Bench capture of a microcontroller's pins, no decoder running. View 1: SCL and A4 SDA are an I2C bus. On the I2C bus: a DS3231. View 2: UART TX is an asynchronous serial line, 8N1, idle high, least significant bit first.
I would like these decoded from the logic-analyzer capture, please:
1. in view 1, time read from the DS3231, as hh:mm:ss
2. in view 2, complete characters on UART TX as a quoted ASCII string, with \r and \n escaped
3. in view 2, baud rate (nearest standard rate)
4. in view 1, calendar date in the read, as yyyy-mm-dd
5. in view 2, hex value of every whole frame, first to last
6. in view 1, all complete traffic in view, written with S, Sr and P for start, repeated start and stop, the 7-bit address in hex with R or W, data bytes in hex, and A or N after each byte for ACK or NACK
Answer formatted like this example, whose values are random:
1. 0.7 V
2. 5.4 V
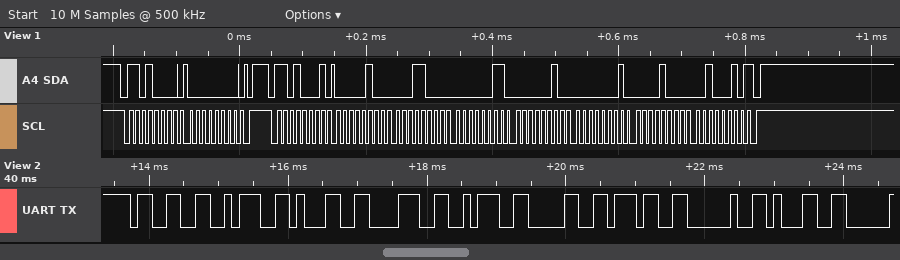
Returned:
1. 03:18:04
2. "3:18:07 1"
3. 9600 baud
4. 2022-08-01
5. 33 3A 31 38 3A 30 37 20 31
6. S 68W A 00 A P S 68R A 04 A 18 A 03 A 02 A 01 A 08 A 22 N P
